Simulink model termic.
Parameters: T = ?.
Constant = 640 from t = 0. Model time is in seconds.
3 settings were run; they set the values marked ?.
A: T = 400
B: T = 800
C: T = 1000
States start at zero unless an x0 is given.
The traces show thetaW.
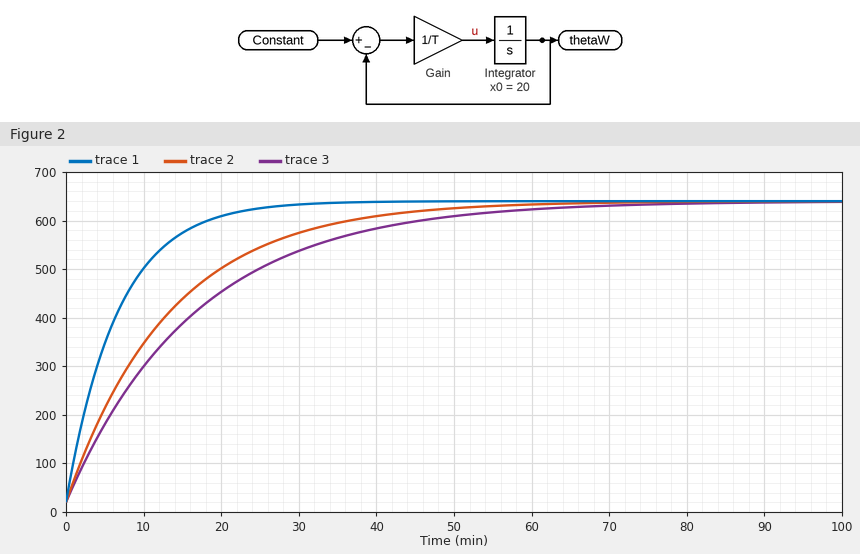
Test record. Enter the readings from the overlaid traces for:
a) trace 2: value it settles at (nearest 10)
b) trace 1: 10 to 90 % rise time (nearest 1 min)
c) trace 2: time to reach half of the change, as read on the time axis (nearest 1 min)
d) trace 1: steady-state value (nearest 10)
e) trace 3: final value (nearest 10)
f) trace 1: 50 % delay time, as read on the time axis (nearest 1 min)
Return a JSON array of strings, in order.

["640", "15 min", "9 min", "640", "640", "5 min"]
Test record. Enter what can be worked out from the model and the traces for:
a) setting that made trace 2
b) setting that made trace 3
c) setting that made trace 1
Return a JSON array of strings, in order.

["B", "C", "A"]
